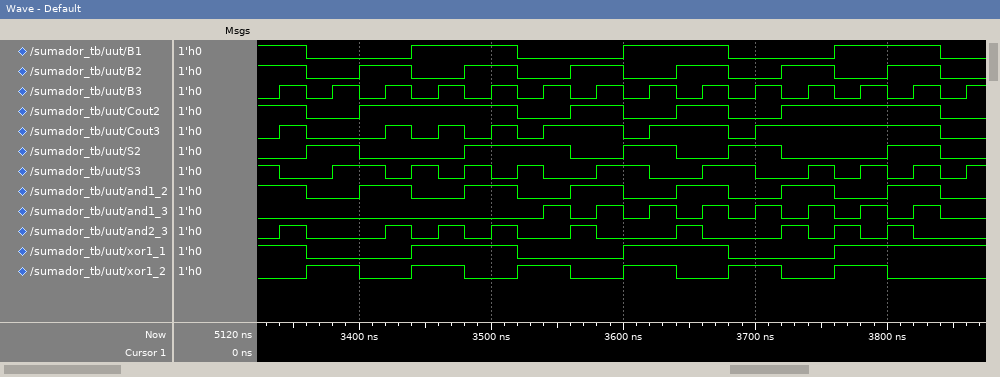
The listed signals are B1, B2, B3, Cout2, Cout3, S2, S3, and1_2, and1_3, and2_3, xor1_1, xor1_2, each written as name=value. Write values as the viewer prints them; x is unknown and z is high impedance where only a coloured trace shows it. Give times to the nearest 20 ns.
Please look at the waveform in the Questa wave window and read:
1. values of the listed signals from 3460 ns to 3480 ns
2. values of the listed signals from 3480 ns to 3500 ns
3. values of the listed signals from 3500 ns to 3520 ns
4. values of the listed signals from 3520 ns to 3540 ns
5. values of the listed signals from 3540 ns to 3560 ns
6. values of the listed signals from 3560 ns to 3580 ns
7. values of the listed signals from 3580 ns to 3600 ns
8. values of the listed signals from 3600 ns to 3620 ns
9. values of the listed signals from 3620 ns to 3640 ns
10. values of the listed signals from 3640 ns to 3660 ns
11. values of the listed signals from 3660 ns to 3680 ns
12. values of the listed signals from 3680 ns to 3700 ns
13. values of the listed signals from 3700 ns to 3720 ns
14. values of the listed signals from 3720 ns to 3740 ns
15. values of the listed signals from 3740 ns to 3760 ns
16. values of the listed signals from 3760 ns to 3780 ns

B1=1, B2=0, B3=1, Cout2=1, Cout3=1, S2=0, S3=0, and1_2=0, and1_3=0, and2_3=1, xor1_1=1, xor1_2=1
B1=1, B2=1, B3=0, Cout2=1, Cout3=0, S2=1, S3=1, and1_2=1, and1_3=0, and2_3=0, xor1_1=1, xor1_2=0
B1=1, B2=1, B3=1, Cout2=1, Cout3=1, S2=1, S3=0, and1_2=1, and1_3=0, and2_3=1, xor1_1=1, xor1_2=0
B1=0, B2=0, B3=0, Cout2=0, Cout3=0, S2=1, S3=1, and1_2=0, and1_3=0, and2_3=0, xor1_1=0, xor1_2=1
B1=0, B2=0, B3=1, Cout2=0, Cout3=1, S2=1, S3=0, and1_2=0, and1_3=1, and2_3=0, xor1_1=0, xor1_2=1
B1=0, B2=1, B3=0, Cout2=1, Cout3=1, S2=0, S3=0, and1_2=1, and1_3=0, and2_3=1, xor1_1=0, xor1_2=0
B1=0, B2=1, B3=1, Cout2=1, Cout3=1, S2=0, S3=1, and1_2=1, and1_3=1, and2_3=0, xor1_1=0, xor1_2=0
B1=1, B2=0, B3=0, Cout2=0, Cout3=0, S2=1, S3=1, and1_2=0, and1_3=0, and2_3=0, xor1_1=1, xor1_2=1
B1=1, B2=0, B3=1, Cout2=0, Cout3=1, S2=1, S3=0, and1_2=0, and1_3=1, and2_3=0, xor1_1=1, xor1_2=1
B1=1, B2=1, B3=0, Cout2=1, Cout3=1, S2=0, S3=0, and1_2=1, and1_3=0, and2_3=1, xor1_1=1, xor1_2=0
B1=1, B2=1, B3=1, Cout2=1, Cout3=1, S2=0, S3=1, and1_2=1, and1_3=1, and2_3=0, xor1_1=1, xor1_2=0
B1=0, B2=0, B3=0, Cout2=0, Cout3=0, S2=1, S3=1, and1_2=0, and1_3=0, and2_3=0, xor1_1=0, xor1_2=1
B1=0, B2=0, B3=1, Cout2=0, Cout3=1, S2=1, S3=0, and1_2=0, and1_3=1, and2_3=0, xor1_1=0, xor1_2=1
B1=0, B2=1, B3=0, Cout2=1, Cout3=1, S2=0, S3=0, and1_2=1, and1_3=0, and2_3=1, xor1_1=0, xor1_2=0
B1=0, B2=1, B3=1, Cout2=1, Cout3=1, S2=0, S3=1, and1_2=1, and1_3=1, and2_3=0, xor1_1=0, xor1_2=0
B1=1, B2=0, B3=0, Cout2=1, Cout3=1, S2=0, S3=0, and1_2=0, and1_3=0, and2_3=1, xor1_1=1, xor1_2=1
